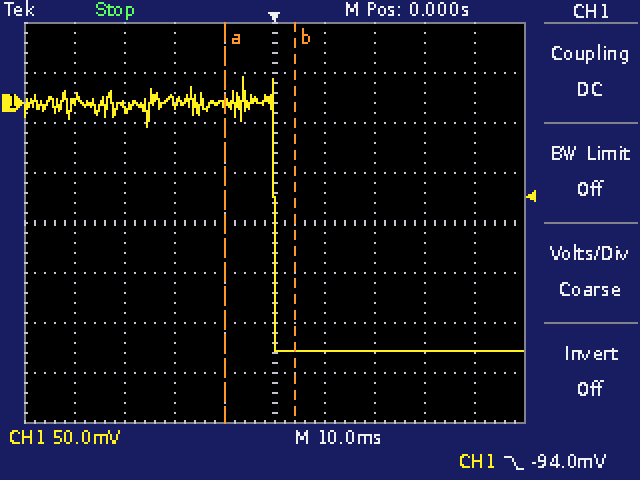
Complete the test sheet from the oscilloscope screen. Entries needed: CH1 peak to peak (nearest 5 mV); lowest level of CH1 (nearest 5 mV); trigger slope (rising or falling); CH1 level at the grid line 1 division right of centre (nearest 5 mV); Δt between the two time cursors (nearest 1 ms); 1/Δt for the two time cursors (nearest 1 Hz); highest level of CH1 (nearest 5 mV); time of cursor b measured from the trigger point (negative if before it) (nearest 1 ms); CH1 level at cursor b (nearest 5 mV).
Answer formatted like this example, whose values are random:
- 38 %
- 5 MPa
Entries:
- 275 mV
- -250 mV
- falling
- -250 mV
- 14 ms
- 71 Hz
- 25 mV
- +4 ms
- -250 mV
